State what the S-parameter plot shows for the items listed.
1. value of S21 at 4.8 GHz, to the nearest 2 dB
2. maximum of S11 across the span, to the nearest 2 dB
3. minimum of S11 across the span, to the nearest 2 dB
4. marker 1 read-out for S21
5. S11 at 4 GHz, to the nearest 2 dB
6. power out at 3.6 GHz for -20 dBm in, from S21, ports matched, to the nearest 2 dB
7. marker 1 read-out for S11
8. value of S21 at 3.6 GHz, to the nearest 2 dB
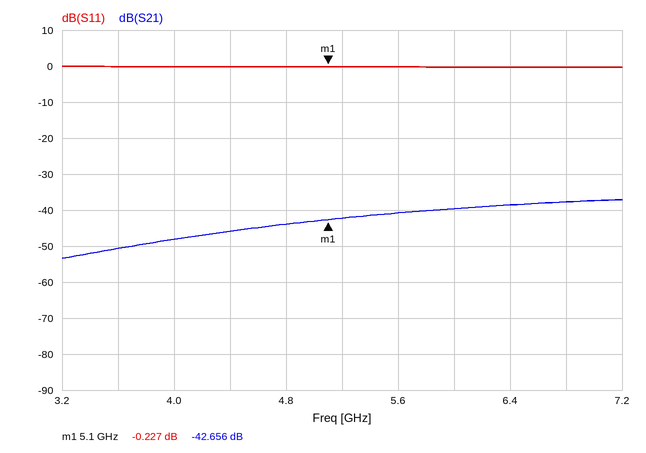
-44 dB
0 dB
0 dB
-42.656 dB
0 dB
-70 dBm
-0.227 dB
-50 dB
